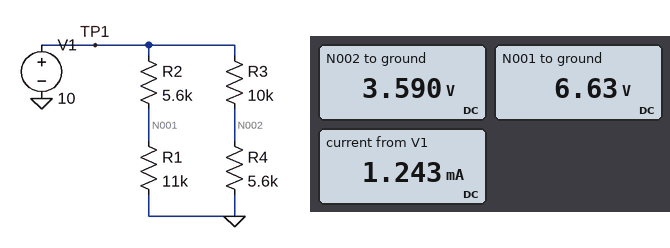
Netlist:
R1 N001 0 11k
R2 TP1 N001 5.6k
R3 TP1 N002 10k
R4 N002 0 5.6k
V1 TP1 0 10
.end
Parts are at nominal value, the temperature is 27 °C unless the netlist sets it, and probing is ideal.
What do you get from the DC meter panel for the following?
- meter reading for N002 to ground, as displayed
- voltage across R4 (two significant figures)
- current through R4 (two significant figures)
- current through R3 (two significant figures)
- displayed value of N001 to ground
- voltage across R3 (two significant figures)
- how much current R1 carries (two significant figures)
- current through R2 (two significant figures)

3.590 V
3.6 V
640 µA
640 µA
6.63 V
6.4 V
600 µA
600 µA
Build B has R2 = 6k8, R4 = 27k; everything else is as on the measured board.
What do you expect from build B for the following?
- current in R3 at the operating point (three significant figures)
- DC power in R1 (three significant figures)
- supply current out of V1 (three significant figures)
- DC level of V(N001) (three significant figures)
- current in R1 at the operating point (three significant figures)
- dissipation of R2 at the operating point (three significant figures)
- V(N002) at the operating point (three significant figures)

270 µA
3.47 mW
832 µA
6.18 V
562 µA
2.15 mW
7.30 V
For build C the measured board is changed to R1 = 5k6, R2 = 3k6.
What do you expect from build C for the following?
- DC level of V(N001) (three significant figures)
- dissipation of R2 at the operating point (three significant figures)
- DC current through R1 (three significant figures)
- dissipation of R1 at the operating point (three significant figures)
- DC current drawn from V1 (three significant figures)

6.09 V
4.25 mW
1.09 mA
6.62 mW
1.73 mA
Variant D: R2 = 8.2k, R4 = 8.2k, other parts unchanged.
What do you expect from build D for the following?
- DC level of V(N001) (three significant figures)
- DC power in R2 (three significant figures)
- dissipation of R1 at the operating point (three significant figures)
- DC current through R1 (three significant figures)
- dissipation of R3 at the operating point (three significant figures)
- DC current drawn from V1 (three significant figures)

5.73 V
2.22 mW
2.98 mW
521 µA
3.02 mW
1.07 mA
